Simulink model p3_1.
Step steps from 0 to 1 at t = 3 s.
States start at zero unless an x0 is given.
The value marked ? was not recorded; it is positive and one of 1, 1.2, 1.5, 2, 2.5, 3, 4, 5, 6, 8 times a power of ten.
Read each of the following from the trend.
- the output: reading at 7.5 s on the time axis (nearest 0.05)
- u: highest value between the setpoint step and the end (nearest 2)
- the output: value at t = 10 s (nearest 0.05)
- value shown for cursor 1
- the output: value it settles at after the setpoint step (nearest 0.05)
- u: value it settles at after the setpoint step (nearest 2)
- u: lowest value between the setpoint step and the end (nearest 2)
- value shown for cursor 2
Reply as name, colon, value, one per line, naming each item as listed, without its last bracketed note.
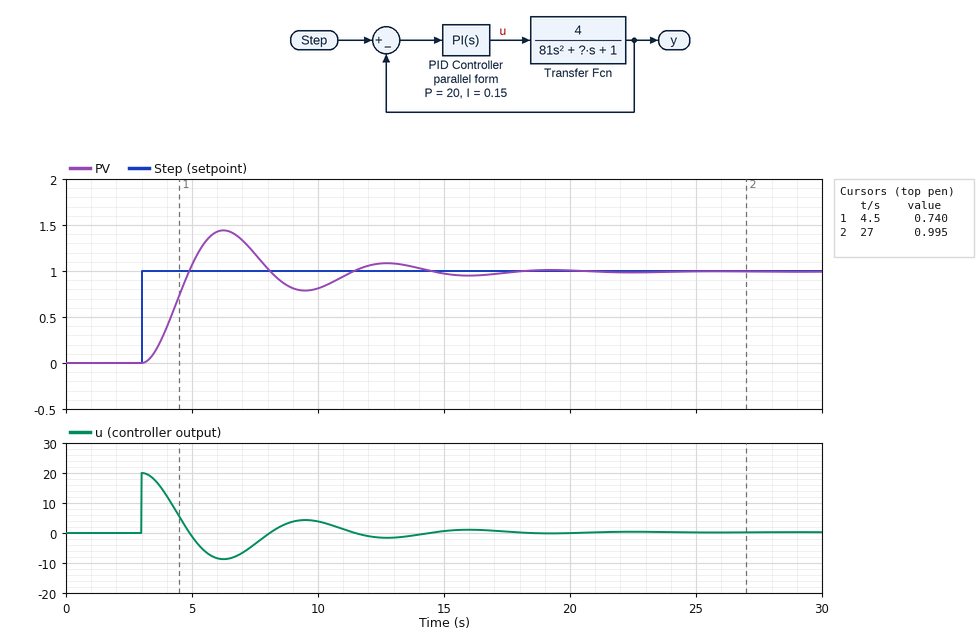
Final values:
the output: reading at 7.5 s on the time axis: 1.20
u: highest value between the setpoint step and the end: 20
the output: value at t = 10 s: 0.80
value shown for cursor 1: 0.740
the output: value it settles at after the setpoint step: 1.00
u: value it settles at after the setpoint step: 0
u: lowest value between the setpoint step and the end: -8
value shown for cursor 2: 0.995
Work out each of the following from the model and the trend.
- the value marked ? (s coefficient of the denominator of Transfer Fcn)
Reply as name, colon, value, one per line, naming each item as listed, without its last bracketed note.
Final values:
the value marked ?: 40
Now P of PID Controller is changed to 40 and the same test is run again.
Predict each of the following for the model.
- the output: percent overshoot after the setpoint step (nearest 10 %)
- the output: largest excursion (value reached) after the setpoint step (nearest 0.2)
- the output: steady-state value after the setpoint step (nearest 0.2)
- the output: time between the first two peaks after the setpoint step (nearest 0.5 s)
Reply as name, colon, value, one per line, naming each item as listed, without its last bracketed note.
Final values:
the output: percent overshoot after the setpoint step: 60 %
the output: largest excursion (value reached) after the setpoint step: 1.6
the output: steady-state value after the setpoint step: 1.0
the output: time between the first two peaks after the setpoint step: 4.5 s
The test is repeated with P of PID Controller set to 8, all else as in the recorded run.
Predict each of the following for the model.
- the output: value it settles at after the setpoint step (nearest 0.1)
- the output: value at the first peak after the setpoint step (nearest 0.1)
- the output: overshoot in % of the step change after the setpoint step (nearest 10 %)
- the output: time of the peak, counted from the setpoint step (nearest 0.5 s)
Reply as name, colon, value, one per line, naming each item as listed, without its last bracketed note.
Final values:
the output: value it settles at after the setpoint step: 1.0
the output: value at the first peak after the setpoint step: 1.3
the output: overshoot in % of the step change after the setpoint step: 30 %
the output: time of the peak, counted from the setpoint step: 5.5 s
